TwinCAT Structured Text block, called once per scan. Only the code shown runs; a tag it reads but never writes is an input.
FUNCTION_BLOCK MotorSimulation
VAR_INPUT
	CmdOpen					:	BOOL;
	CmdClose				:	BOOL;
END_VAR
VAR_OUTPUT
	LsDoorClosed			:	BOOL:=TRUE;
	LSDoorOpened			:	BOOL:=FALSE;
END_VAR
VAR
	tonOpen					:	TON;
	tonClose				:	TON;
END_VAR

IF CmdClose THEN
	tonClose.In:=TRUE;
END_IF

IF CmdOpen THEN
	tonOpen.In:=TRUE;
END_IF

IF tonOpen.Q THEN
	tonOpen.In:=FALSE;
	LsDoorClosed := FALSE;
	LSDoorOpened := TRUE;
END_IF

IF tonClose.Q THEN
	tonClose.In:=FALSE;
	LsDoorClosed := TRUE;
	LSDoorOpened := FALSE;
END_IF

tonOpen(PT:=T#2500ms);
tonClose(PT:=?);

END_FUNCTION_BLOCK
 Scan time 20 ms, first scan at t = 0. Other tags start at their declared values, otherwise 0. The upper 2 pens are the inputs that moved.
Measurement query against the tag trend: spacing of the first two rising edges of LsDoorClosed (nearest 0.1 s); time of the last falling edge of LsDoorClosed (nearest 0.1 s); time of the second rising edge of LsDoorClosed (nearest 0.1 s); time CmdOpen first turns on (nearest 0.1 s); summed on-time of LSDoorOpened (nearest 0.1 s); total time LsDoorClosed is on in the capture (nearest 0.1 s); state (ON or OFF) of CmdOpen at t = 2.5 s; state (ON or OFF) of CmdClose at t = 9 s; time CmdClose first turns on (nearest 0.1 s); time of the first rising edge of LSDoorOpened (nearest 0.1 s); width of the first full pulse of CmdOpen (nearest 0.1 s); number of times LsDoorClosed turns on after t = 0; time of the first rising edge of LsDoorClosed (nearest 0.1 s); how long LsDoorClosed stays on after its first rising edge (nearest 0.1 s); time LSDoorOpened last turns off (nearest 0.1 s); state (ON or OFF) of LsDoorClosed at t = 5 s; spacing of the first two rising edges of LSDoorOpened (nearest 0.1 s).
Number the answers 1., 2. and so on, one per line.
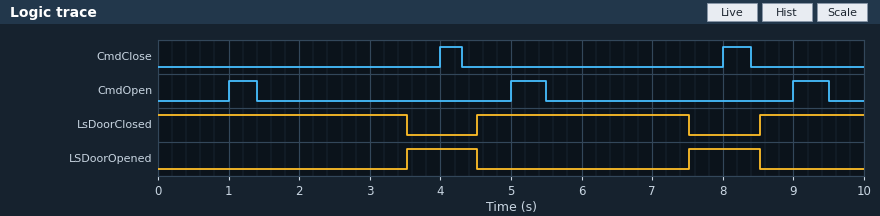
1. 4.0 s
2. 7.5 s
3. 8.5 s
4. 1.0 s
5. 2.0 s
6. 8.0 s
7. OFF
8. OFF
9. 4.0 s
10. 3.5 s
11. 0.4 s
12. 2
13. 4.5 s
14. 3.0 s
15. 8.5 s
16. ON
17. 4.0 s
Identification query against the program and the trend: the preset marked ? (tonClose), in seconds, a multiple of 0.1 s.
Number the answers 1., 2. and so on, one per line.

1. 0.5 s
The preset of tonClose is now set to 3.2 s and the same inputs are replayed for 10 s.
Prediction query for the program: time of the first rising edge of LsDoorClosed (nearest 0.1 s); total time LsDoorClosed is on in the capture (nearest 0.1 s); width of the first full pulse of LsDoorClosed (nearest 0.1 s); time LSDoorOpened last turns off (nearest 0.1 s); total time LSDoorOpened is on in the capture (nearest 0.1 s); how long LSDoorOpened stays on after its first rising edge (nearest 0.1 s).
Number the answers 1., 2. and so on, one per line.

1. 7.2 s
2. 3.8 s
3. 0.3 s
4. 7.2 s
5. 6.2 s
6. 3.7 s
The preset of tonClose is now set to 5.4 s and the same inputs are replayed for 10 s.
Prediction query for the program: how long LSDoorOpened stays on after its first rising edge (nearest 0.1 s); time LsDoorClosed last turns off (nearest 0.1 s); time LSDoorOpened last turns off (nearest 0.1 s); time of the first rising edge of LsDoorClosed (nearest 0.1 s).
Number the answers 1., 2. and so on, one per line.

1. 5.9 s
2. 3.5 s
3. 9.4 s
4. 9.4 s
